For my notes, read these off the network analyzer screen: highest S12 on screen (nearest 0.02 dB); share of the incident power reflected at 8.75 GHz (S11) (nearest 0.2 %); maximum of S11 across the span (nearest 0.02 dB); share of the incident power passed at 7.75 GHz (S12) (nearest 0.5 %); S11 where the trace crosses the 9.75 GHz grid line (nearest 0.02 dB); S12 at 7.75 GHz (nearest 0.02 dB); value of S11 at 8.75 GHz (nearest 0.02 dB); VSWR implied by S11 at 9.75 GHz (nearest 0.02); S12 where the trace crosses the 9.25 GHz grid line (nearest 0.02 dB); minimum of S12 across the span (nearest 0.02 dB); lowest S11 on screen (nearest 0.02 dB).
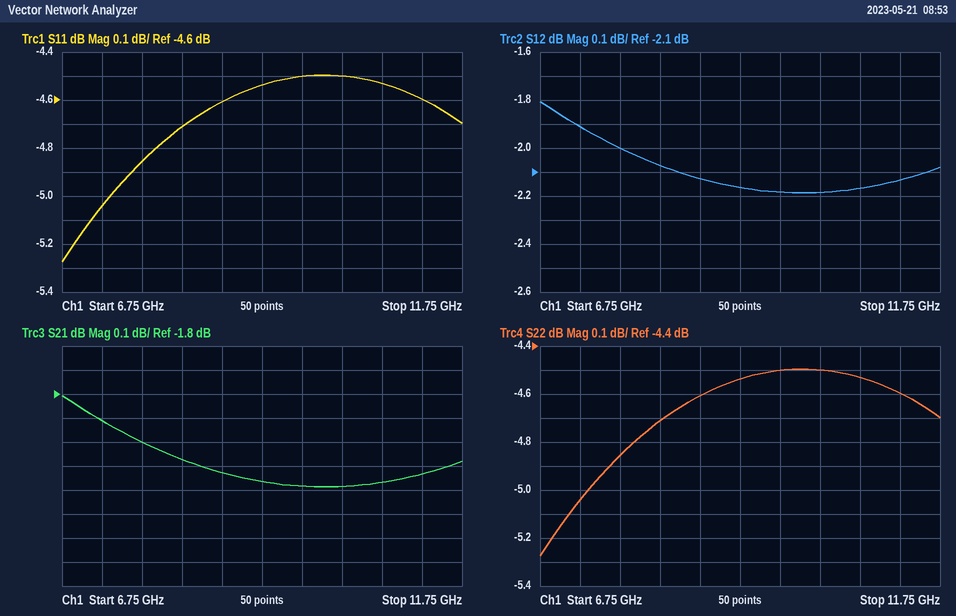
-1.80 dB
34.6 %
-4.50 dB
63.0 %
-4.50 dB
-2.00 dB
-4.60 dB
3.94
-2.16 dB
-2.18 dB
-5.28 dB
